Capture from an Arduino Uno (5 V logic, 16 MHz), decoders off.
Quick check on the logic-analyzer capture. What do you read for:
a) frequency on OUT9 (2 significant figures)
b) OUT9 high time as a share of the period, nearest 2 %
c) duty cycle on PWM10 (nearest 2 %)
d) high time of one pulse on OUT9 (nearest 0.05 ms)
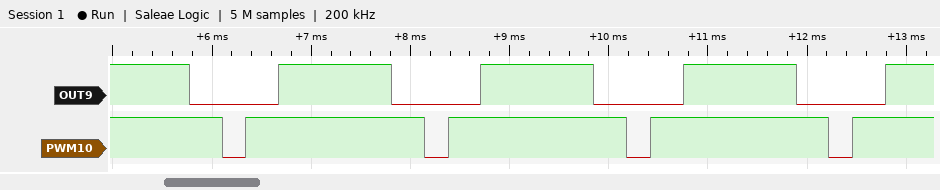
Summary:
490 Hz
56 %
88 %
1.15 ms
